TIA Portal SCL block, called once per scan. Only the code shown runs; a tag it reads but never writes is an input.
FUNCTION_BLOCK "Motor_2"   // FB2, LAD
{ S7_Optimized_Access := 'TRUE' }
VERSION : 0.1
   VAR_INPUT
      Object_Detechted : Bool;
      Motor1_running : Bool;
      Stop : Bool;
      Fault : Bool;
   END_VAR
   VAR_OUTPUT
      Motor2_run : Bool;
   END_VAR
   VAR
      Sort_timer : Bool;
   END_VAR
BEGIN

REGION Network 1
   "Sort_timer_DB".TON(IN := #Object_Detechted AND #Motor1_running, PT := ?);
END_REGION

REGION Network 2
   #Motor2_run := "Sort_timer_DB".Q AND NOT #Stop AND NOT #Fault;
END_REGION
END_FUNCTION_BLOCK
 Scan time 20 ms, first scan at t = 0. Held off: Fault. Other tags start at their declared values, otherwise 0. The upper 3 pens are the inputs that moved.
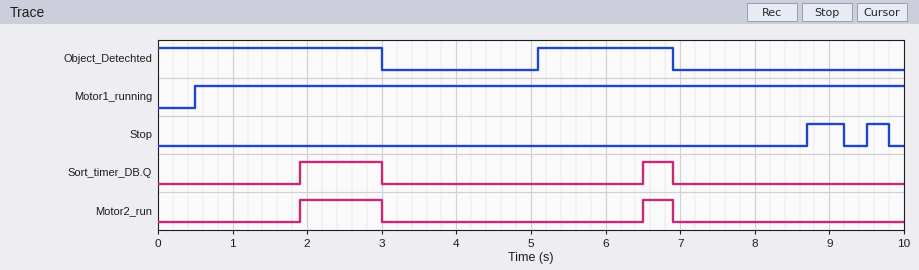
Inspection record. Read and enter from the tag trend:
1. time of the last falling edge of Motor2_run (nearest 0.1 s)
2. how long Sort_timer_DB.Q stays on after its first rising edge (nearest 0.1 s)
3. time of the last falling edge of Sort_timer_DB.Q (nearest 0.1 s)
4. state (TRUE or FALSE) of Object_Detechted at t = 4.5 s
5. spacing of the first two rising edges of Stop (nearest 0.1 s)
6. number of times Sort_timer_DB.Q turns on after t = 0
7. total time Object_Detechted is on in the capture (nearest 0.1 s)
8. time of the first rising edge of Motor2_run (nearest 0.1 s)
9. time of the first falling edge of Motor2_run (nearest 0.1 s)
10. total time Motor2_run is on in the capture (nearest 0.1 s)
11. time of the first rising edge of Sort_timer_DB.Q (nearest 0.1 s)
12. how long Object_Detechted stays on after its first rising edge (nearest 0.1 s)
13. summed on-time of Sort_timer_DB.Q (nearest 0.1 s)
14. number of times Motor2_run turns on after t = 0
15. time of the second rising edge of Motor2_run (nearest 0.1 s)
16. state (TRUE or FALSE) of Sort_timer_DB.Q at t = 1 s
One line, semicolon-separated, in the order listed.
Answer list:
6.9 s; 1.1 s; 6.9 s; FALSE; 0.8 s; 2; 4.8 s; 1.9 s; 3.0 s; 1.5 s; 1.9 s; 1.8 s; 1.5 s; 2; 6.5 s; FALSE
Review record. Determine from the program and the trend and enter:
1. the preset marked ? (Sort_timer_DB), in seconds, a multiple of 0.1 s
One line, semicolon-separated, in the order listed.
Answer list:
1.4 s
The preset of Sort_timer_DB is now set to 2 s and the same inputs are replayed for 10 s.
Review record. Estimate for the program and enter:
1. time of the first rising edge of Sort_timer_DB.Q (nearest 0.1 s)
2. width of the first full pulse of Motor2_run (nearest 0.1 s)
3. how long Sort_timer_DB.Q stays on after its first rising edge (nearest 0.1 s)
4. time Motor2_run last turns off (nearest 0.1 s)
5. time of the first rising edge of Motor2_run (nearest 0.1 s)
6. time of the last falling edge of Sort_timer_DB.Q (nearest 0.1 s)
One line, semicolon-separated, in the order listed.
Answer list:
2.5 s; 0.5 s; 0.5 s; 3.0 s; 2.5 s; 3.0 s
